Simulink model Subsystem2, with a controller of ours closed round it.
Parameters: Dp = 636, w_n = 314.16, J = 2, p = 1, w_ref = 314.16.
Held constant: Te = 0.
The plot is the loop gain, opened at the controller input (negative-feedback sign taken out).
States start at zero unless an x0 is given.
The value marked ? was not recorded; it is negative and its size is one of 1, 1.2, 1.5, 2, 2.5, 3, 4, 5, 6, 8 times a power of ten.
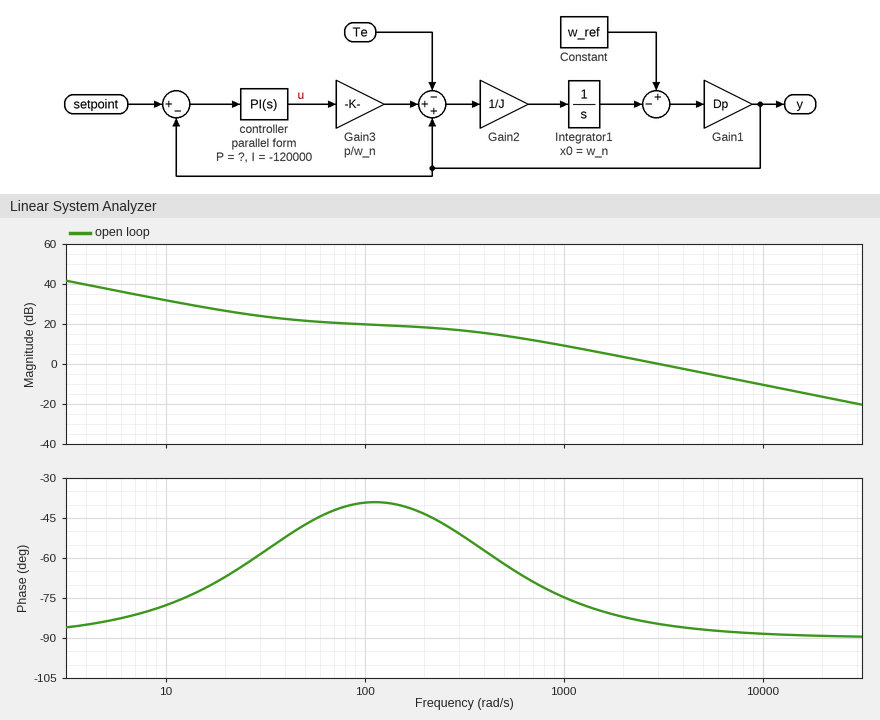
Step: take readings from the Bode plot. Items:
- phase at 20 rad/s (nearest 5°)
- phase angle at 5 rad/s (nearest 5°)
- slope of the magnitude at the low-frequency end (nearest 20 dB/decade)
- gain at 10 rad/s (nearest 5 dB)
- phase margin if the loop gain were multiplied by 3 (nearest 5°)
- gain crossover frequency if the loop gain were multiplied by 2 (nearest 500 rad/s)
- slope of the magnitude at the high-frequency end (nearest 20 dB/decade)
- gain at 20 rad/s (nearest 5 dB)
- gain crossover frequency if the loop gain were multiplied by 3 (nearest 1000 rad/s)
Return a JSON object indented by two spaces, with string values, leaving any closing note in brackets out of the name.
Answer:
{
  "phase at 20 rad/s": "-65°",
  "phase angle at 5 rad/s": "-85°",
  "slope of the magnitude at the low-frequency end": "-20 dB/decade",
  "gain at 10 rad/s": "30 dB",
  "phase margin if the loop gain were multiplied by 3": "90°",
  "gain crossover frequency if the loop gain were multiplied by 2": "6000 rad/s",
  "slope of the magnitude at the high-frequency end": "-20 dB/decade",
  "gain at 20 rad/s": "25 dB",
  "gain crossover frequency if the loop gain were multiplied by 3": "9000 rad/s"
}
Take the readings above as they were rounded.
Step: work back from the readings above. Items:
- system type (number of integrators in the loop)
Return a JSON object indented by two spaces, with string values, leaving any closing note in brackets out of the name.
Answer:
{
  "system type": "1"
}
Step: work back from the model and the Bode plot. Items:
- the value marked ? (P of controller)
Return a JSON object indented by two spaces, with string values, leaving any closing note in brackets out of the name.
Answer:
{
  "the value marked ?": "-3000"
}
